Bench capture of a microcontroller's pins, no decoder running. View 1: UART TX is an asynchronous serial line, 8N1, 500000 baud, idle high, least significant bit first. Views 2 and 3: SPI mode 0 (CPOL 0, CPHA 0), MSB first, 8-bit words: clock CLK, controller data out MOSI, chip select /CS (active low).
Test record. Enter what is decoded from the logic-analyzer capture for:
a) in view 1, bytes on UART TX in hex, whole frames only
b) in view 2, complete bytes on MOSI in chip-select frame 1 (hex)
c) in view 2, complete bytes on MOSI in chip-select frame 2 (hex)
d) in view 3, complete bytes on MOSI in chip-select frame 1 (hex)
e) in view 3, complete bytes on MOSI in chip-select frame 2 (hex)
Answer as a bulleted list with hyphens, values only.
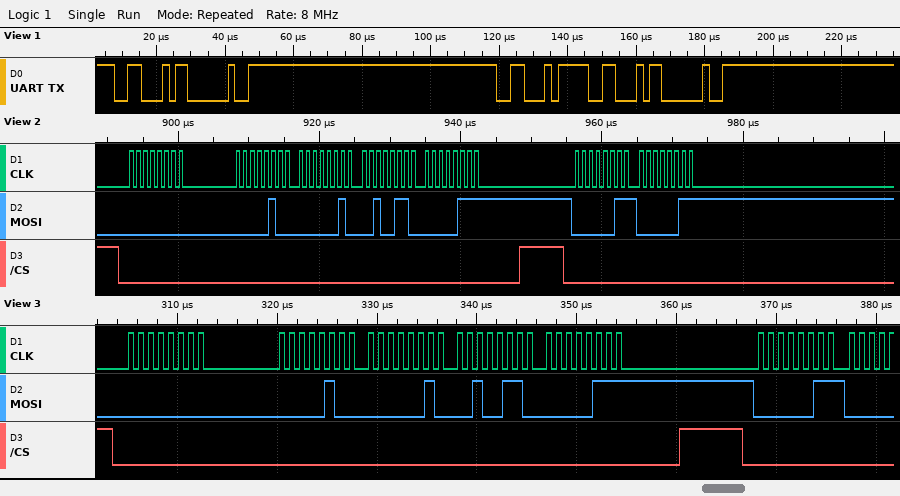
- 46 20 46 46 20
- 0x00 0x04 0x02 0x26 0x07
- 0x03 0x03
- 0x00 0x04 0x02 0x26 0x07
- 0x03
